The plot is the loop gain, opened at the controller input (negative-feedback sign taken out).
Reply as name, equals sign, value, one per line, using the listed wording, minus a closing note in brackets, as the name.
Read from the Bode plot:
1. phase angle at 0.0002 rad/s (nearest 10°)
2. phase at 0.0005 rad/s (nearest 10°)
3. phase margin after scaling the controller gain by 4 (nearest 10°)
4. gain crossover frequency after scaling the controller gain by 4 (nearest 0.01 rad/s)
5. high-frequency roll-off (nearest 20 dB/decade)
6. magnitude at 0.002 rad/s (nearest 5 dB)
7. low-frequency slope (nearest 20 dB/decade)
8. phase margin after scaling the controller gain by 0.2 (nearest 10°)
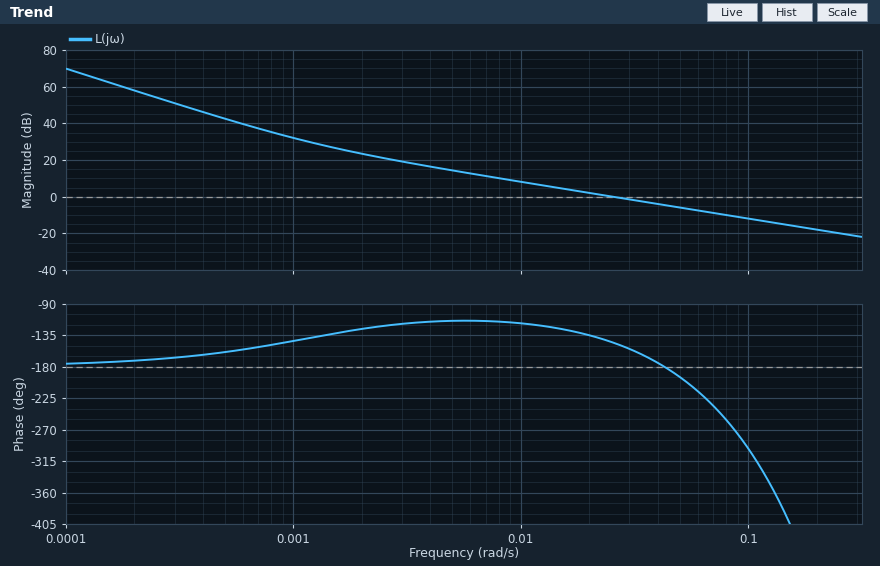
phase angle at 0.0002 rad/s = -170°
phase at 0.0005 rad/s = -160°
phase margin after scaling the controller gain by 4 = -120°
gain crossover frequency after scaling the controller gain by 4 = 0.10 rad/s
high-frequency roll-off = -20 dB/decade
magnitude at 0.002 rad/s = 25 dB
low-frequency slope = -40 dB/decade
phase margin after scaling the controller gain by 0.2 = 70°
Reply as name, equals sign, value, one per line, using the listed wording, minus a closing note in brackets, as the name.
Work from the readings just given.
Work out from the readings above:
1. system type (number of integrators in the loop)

system type = 2
